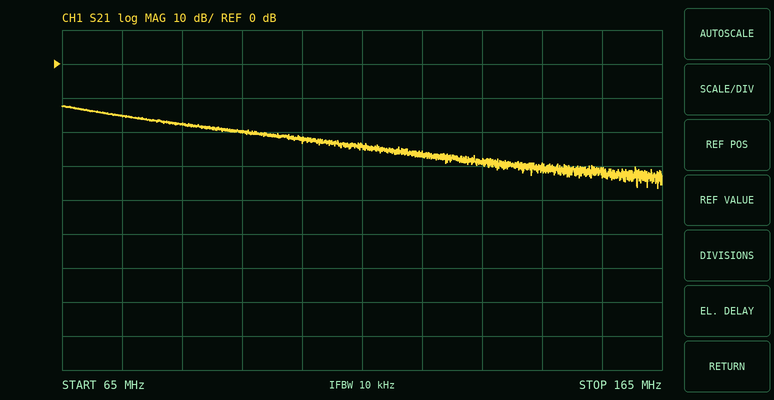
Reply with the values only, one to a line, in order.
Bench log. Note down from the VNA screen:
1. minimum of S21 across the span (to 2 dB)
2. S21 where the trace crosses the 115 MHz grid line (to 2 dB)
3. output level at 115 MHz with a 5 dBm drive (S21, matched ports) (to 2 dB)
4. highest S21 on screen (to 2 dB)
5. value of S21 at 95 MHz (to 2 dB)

-36 dB
-24 dB
-18 dBm
-12 dB
-20 dB
